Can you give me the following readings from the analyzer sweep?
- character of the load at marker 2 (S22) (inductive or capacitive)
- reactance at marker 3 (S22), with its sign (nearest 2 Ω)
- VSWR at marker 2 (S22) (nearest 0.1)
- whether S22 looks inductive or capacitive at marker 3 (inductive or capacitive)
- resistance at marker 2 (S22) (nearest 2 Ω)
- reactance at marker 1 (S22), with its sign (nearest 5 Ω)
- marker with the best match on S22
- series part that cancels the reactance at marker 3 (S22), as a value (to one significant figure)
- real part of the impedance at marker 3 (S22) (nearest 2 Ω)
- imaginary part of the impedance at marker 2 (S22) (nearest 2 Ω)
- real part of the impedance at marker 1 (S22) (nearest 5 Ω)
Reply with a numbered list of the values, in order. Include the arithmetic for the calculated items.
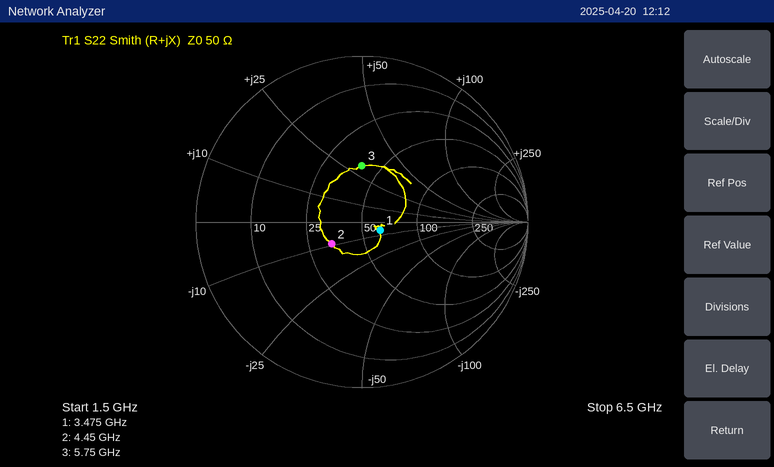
1. capacitive
2. +30 Ω
3. 1.6
4. inductive
5. 34 Ω
6. -5 Ω
7. marker 1
8. C = 1/(2π × 5.75 GHz × 30 Ω) ≈ 923 fF, so 900 fF to one significant figure
9. 40 Ω
10. -10 Ω
11. 60 Ω
